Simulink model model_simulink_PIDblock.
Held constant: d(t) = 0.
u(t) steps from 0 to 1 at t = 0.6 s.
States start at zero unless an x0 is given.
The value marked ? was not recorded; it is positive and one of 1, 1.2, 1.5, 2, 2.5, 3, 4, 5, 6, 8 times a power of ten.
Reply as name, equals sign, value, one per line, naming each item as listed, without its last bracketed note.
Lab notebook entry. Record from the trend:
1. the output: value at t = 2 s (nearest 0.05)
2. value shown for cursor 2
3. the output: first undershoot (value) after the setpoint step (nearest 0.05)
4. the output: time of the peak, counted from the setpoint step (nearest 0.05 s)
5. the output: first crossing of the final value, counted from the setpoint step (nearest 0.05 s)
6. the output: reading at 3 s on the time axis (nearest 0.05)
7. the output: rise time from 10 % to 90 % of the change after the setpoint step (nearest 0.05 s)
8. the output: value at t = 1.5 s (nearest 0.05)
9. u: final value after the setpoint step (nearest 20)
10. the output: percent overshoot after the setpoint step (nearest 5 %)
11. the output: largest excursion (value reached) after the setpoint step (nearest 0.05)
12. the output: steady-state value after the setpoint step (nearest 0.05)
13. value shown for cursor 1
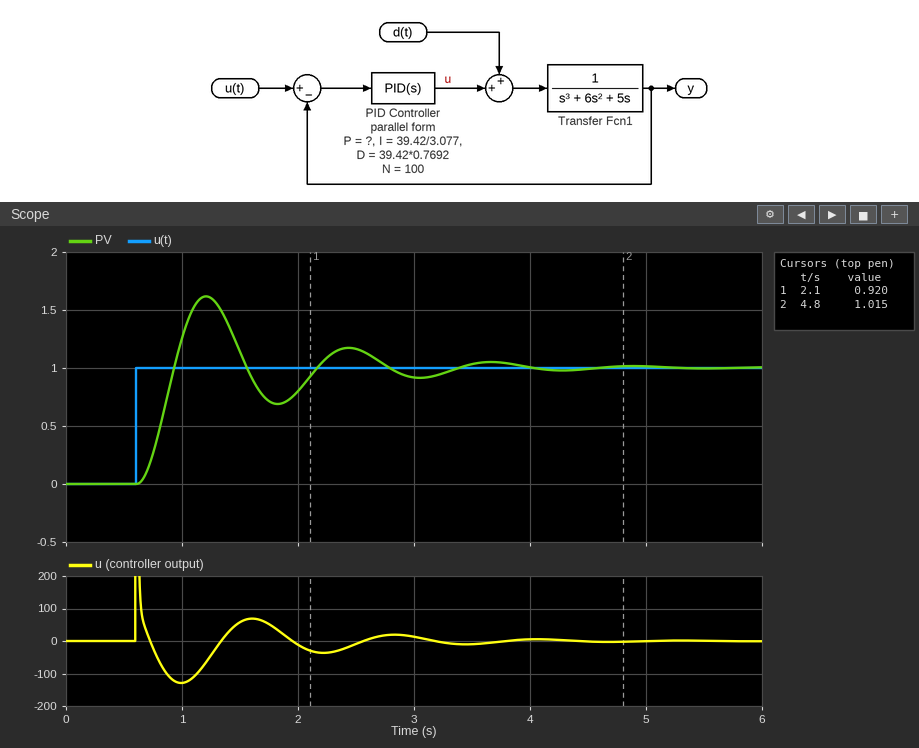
the output: value at t = 2 s = 0.80
value shown for cursor 2 = 1.015
the output: first undershoot (value) after the setpoint step = 0.70
the output: time of the peak, counted from the setpoint step = 0.60 s
the output: first crossing of the final value, counted from the setpoint step = 0.35 s
the output: reading at 3 s on the time axis = 0.90
the output: rise time from 10 % to 90 % of the change after the setpoint step = 0.20 s
the output: value at t = 1.5 s = 1.15
u: final value after the setpoint step = 0
the output: percent overshoot after the setpoint step = 60 %
the output: largest excursion (value reached) after the setpoint step = 1.60
the output: steady-state value after the setpoint step = 1.00
value shown for cursor 1 = 0.920
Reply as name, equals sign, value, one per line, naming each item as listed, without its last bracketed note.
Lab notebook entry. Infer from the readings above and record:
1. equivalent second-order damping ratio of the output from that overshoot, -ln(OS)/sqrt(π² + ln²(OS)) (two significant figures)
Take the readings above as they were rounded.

equivalent second-order damping ratio of the output from that overshoot, -ln(OS)/sqrt(π² + ln²(OS)) = 0.16
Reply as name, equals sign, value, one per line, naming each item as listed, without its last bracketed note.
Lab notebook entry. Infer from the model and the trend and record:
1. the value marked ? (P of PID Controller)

the value marked ? = 100
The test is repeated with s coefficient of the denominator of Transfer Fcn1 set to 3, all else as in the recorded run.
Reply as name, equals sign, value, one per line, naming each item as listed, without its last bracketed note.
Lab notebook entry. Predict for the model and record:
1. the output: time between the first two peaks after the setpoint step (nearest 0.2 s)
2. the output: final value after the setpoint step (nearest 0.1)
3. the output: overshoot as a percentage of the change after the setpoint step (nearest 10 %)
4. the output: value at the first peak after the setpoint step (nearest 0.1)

the output: time between the first two peaks after the setpoint step = 1.2 s
the output: final value after the setpoint step = 1.0
the output: overshoot as a percentage of the change after the setpoint step = 70 %
the output: value at the first peak after the setpoint step = 1.7
